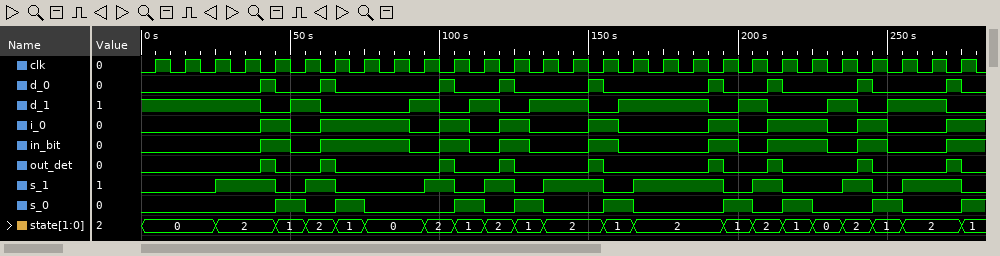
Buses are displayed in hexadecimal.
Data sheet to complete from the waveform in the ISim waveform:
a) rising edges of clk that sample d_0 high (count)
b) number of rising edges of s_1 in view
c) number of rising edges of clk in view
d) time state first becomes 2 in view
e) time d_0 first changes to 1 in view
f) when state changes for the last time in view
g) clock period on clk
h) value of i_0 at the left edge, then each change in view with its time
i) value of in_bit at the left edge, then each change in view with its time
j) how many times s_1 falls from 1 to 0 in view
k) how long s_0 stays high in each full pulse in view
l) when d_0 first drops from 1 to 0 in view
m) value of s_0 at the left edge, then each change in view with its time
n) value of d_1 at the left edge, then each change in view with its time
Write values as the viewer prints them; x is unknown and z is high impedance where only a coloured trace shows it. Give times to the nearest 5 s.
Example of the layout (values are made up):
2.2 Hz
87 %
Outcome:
9
9
28
25 s
40 s
275 s
10 s
0, 1 at 40 s, 0 at 50 s, 1 at 60 s, 0 at 90 s, 1 at 100 s, 0 at 110 s, 1 at 120 s, 0 at 130 s, 1 at 150 s, 0 at 160 s, 1 at 190 s, 0 at 200 s, 1 at 210 s, 0 at 230 s, 1 at 240 s, 0 at 250 s, 1 at 270 s
0, 1 at 40 s, 0 at 50 s, 1 at 60 s, 0 at 90 s, 1 at 100 s, 0 at 110 s, 1 at 120 s, 0 at 130 s, 1 at 150 s, 0 at 160 s, 1 at 190 s, 0 at 200 s, 1 at 210 s, 0 at 230 s, 1 at 240 s, 0 at 250 s, 1 at 270 s
9
10 s, 10 s, 10 s, 10 s, 10 s, 10 s, 10 s, 10 s
45 s
0, 1 at 45 s, 0 at 55 s, 1 at 65 s, 0 at 75 s, 1 at 105 s, 0 at 115 s, 1 at 125 s, 0 at 135 s, 1 at 155 s, 0 at 165 s, 1 at 195 s, 0 at 205 s, 1 at 215 s, 0 at 225 s, 1 at 245 s, 0 at 255 s, 1 at 275 s
1, 0 at 40 s, 1 at 50 s, 0 at 60 s, 1 at 90 s, 0 at 100 s, 1 at 110 s, 0 at 120 s, 1 at 130 s, 0 at 150 s, 1 at 160 s, 0 at 190 s, 1 at 200 s, 0 at 210 s, 1 at 230 s, 0 at 240 s, 1 at 250 s, 0 at 270 s
